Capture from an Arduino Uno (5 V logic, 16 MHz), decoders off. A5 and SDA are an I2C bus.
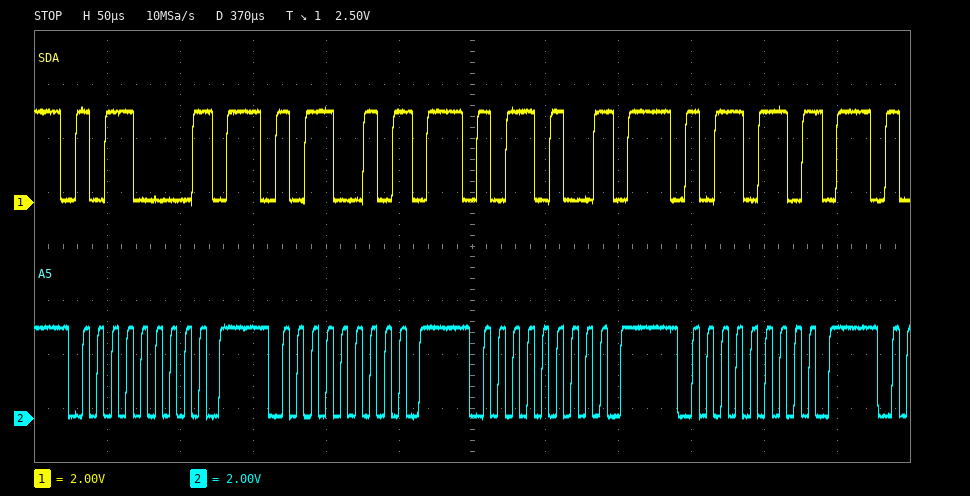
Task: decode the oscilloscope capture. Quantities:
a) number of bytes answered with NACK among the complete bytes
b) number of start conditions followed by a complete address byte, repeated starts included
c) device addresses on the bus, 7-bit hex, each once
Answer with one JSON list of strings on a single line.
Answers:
["4", "4", "0x58 0x59 0x5A 0x5B"]
